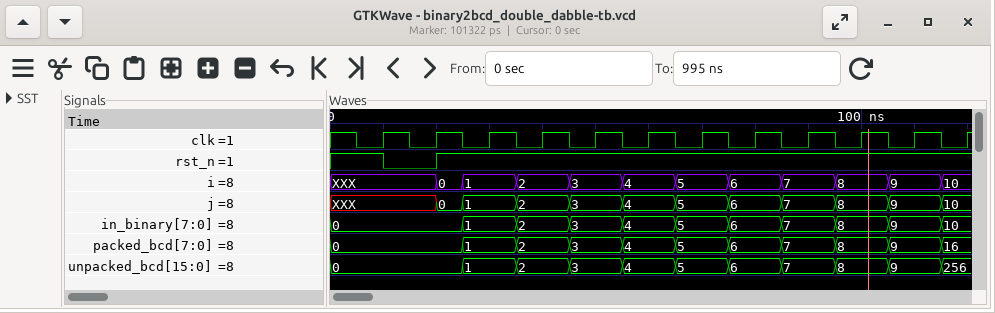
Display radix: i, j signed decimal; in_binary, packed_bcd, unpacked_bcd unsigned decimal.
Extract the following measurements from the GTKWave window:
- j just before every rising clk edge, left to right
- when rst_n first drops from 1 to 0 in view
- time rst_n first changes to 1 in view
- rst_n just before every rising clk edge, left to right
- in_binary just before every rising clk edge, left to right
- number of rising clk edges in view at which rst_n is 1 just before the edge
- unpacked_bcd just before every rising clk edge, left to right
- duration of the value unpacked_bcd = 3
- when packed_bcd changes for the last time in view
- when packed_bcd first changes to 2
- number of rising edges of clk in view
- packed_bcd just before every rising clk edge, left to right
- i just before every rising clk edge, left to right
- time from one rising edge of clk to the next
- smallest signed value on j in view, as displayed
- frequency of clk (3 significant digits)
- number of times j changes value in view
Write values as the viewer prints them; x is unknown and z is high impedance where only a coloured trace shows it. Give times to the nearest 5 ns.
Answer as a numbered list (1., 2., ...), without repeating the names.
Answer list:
1. XXX, XXX, 1, 2, 3, 4, 5, 6, 7, 8, 9, 10
2. 10 ns
3. 20 ns
4. 1 0 1 1 1 1 1 1 1 1 1 1
5. 0, 0, 1, 2, 3, 4, 5, 6, 7, 8, 9, 10
6. 11
7. 0, 0, 1, 2, 3, 4, 5, 6, 7, 8, 9, 256
8. 10 ns
9. 115 ns
10. 35 ns
11. 12
12. 0, 0, 1, 2, 3, 4, 5, 6, 7, 8, 9, 16
13. XXX, XXX, 1, 2, 3, 4, 5, 6, 7, 8, 9, 10
14. 10 ns
15. 0
16. 100 MHz
17. 11
